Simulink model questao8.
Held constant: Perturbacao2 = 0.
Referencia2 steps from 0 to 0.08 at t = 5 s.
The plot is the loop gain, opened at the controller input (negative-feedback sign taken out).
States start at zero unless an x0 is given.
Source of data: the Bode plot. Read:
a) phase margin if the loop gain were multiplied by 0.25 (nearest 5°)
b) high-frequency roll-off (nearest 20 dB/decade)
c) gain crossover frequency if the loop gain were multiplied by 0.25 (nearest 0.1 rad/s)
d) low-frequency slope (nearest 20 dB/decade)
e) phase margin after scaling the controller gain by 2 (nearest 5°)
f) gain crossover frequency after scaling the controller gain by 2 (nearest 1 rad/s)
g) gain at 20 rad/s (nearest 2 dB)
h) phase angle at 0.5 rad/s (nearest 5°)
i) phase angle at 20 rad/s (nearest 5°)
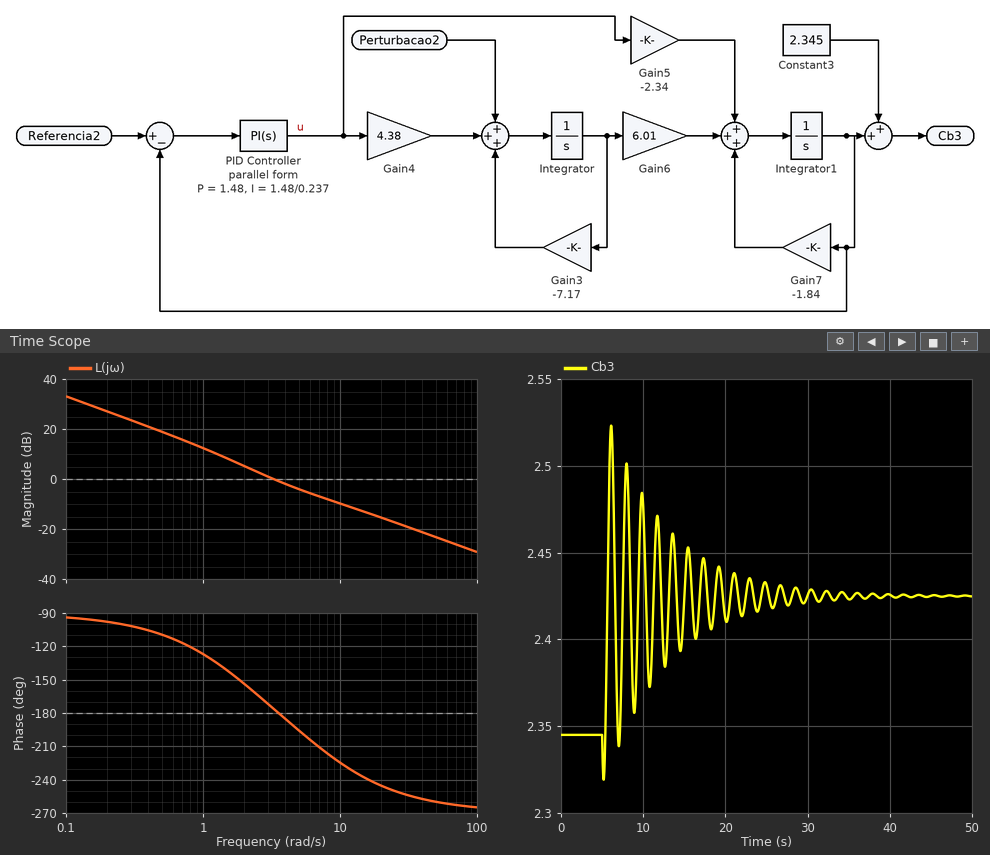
50°
-20 dB/decade
1.0 rad/s
-20 dB/decade
-25°
6 rad/s
-16 dB
-110°
-245°
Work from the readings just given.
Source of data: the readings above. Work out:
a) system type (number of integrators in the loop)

1
